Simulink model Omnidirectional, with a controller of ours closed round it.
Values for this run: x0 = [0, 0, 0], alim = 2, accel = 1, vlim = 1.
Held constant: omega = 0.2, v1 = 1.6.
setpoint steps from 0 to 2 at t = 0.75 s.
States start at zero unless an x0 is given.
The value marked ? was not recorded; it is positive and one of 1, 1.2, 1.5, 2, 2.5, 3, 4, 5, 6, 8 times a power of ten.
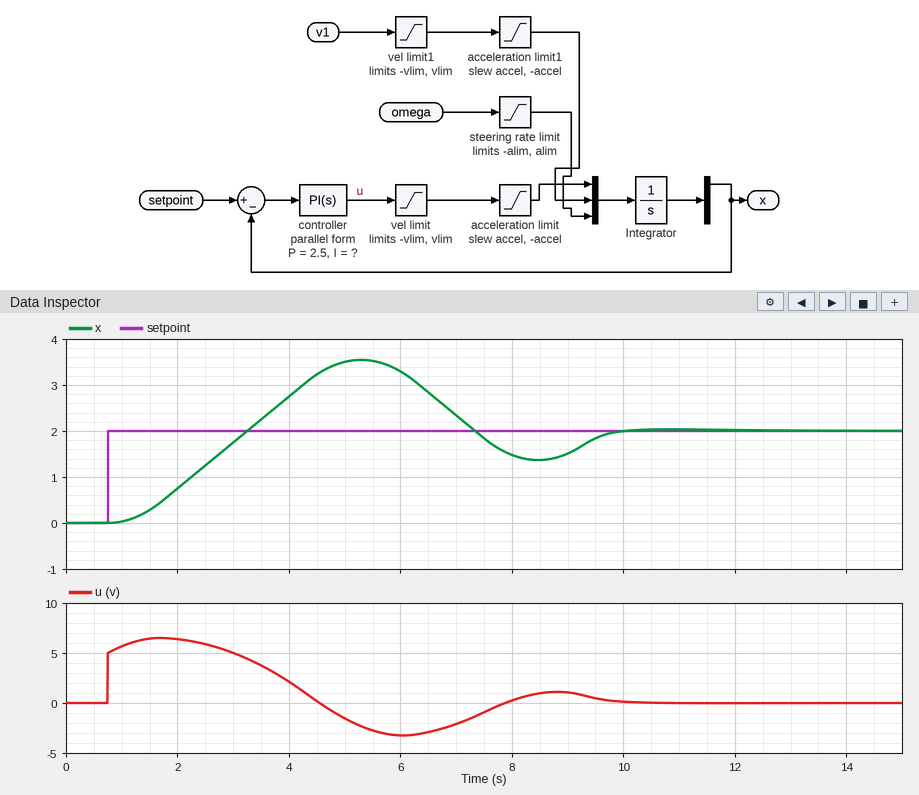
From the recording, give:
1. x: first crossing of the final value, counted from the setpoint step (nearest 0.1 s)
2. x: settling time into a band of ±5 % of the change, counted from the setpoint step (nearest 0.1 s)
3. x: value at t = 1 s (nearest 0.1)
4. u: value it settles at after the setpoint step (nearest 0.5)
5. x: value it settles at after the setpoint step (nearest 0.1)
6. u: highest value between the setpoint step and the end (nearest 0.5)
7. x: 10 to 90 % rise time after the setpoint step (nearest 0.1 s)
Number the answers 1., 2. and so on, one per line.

1. 2.5 s
2. 8.9 s
3. 0.0
4. 0.0
5. 2.0
6. 6.5
7. 1.7 s
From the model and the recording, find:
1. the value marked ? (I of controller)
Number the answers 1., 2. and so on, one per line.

1. 1.5
